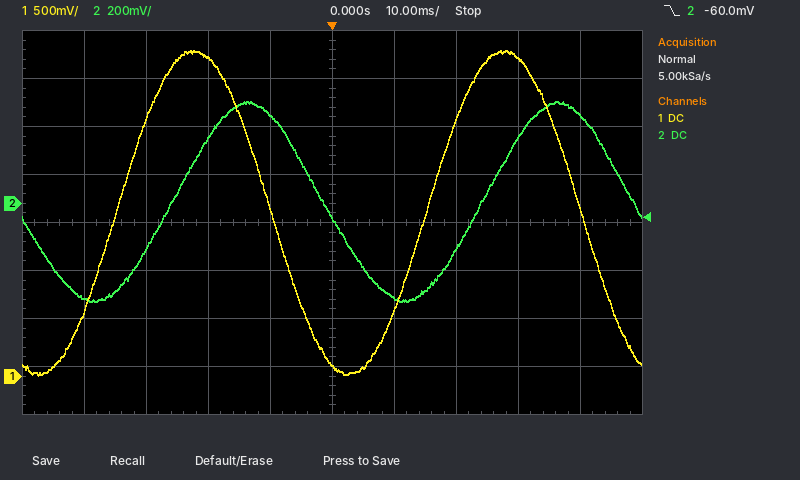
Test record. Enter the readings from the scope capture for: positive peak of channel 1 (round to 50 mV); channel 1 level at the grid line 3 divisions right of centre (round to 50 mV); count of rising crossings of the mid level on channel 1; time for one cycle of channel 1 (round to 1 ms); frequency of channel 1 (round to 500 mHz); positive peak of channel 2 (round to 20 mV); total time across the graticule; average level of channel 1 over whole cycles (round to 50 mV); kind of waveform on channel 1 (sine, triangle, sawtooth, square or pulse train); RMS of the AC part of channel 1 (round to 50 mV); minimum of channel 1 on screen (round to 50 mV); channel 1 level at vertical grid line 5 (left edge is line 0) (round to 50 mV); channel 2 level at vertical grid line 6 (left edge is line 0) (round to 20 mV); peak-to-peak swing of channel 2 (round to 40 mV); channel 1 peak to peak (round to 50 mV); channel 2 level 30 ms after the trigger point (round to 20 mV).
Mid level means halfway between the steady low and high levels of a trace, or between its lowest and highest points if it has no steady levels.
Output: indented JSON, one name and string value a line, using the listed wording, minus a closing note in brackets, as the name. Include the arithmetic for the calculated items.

{
  "positive peak of channel 1": "3.40 V",
  "channel 1 level at the grid line 3 divisions right of centre": "3.30 V",
  "count of rising crossings of the mid level on channel 1": "2",
  "time for one cycle of channel 1": "50 ms",
  "frequency of channel 1": "1 / 50 ms ≈ 20.0 Hz",
  "positive peak of channel 2": "420 mV",
  "total time across the graticule": "100 ms",
  "average level of channel 1 over whole cycles": "(3.40 V + (0 mV)) / 2 ≈ 1.70 V",
  "kind of waveform on channel 1": "sine",
  "RMS of the AC part of channel 1": "3.40 V / (2√2) ≈ 1.20 V",
  "minimum of channel 1 on screen": "0 mV",
  "channel 1 level at vertical grid line 5 (left edge is line 0)": "100 mV",
  "channel 2 level at vertical grid line 6 (left edge is line 0)": "-400 mV",
  "peak-to-peak swing of channel 2": "840 mV",
  "channel 1 peak to peak": "3.40 V − (0 mV) = 3.40 V",
  "channel 2 level 30 ms after the trigger point": "280 mV"
}
